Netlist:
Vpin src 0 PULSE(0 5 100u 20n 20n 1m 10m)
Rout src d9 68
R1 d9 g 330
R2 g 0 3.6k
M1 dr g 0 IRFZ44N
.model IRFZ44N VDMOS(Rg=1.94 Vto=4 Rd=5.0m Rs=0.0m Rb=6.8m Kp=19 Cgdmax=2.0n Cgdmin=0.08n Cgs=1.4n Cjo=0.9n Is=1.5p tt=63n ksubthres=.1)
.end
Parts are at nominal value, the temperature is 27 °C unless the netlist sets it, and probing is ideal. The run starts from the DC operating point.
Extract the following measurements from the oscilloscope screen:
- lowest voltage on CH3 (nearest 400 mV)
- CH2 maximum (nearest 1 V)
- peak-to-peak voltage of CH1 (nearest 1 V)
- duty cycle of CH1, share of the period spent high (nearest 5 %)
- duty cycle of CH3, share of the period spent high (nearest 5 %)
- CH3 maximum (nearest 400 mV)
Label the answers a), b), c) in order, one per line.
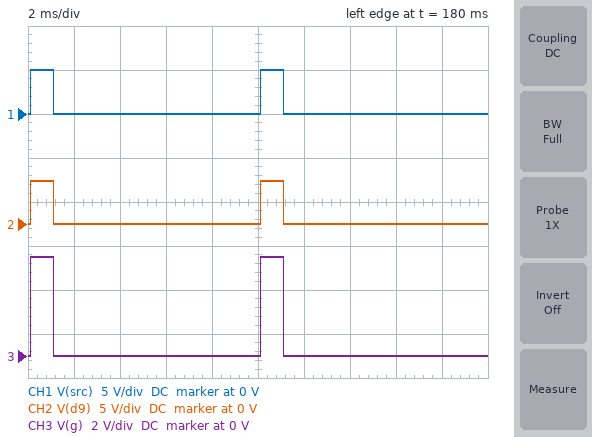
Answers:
a) 0 V
b) 5 V
c) 5 V
d) 10 %
e) 10 %
f) 4.4 V
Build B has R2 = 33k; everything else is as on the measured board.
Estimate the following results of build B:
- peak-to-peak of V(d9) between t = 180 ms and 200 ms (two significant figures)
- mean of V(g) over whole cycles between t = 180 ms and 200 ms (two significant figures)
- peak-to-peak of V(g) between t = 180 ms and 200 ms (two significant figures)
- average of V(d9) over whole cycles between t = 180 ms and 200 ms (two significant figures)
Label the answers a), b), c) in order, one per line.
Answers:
a) 5.0 V
b) 490 mV
c) 4.9 V
d) 500 mV
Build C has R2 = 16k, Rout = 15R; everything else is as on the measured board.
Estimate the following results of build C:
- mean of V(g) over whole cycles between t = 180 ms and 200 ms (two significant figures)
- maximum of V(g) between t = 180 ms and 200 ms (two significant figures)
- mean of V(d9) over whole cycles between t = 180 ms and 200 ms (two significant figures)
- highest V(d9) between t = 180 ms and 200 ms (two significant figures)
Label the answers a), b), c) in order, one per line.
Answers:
a) 490 mV
b) 4.9 V
c) 500 mV
d) 5.0 V
